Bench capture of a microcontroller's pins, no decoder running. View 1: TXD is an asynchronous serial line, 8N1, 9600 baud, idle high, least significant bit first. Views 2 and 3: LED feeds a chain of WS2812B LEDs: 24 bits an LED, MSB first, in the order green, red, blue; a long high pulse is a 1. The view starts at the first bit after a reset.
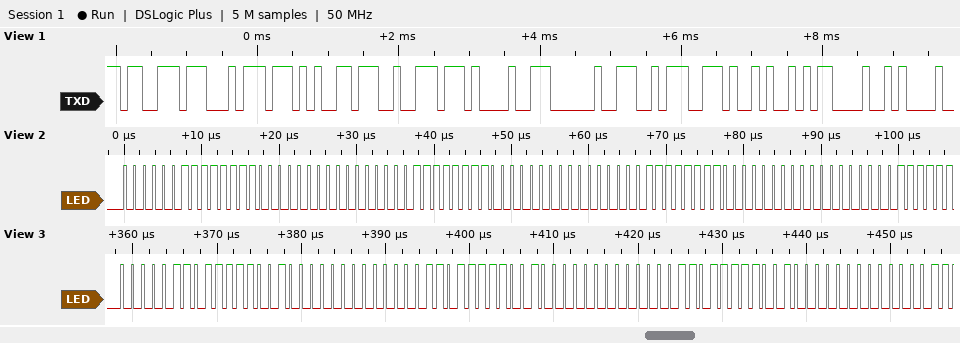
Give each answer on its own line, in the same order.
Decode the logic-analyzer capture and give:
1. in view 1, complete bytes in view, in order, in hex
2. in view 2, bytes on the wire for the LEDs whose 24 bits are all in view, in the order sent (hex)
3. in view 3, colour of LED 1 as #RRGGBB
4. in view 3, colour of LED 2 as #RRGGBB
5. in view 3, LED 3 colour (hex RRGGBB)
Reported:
0x73 0x74 0x65 0x72 0x21 0x20 0x3A 0x29 0x0D 0x0A
03 FC 00 03 FC 00 03 FC 00
#F90600
#F90600
#F90600
